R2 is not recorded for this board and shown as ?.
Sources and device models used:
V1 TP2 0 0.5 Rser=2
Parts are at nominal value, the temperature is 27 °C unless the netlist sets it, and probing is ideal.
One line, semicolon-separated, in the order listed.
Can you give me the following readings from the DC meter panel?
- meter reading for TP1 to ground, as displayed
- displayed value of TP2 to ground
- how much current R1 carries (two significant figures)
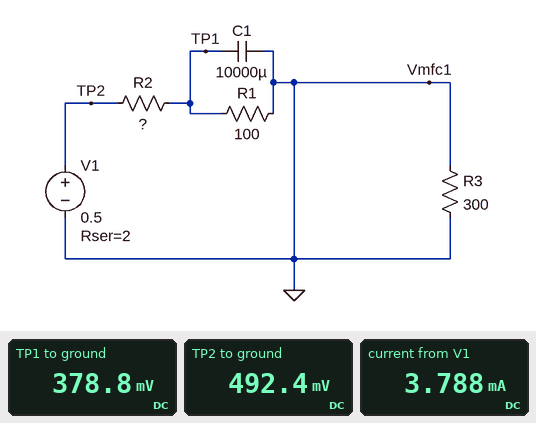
378.8 mV; 492.4 mV; 3.8 mA
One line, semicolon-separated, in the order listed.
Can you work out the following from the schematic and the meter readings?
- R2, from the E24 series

30 Ω
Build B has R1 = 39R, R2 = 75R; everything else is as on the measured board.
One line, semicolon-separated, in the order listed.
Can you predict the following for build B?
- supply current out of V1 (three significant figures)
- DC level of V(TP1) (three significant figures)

4.31 mA; 168 mV
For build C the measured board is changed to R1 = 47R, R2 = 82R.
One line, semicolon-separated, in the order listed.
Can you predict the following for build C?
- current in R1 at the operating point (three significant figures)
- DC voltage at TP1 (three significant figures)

3.82 mA; 179 mV
